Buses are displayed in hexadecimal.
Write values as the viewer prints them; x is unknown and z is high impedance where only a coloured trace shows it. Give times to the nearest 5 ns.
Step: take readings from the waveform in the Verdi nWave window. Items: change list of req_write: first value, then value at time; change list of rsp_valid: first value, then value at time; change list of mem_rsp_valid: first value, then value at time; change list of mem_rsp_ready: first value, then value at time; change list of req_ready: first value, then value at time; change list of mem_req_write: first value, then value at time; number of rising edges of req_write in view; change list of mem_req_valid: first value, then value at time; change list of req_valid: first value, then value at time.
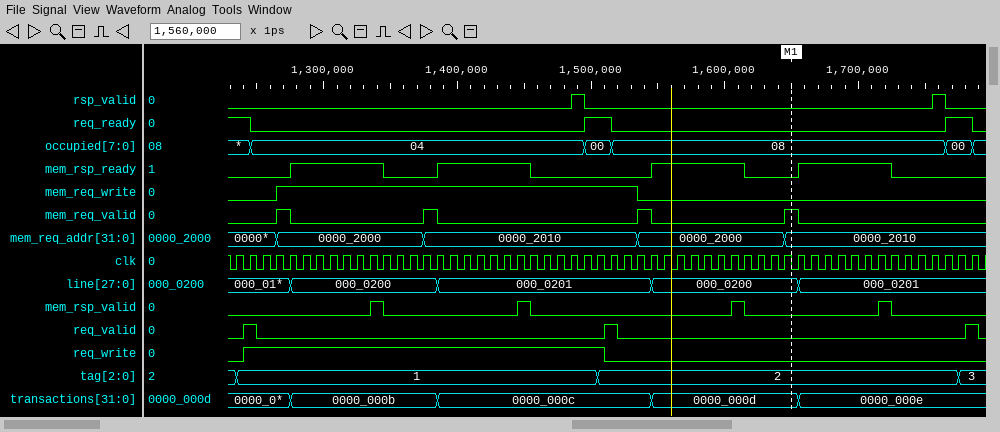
0, 1 at 1240 ns, 0 at 1510 ns
0, 1 at 1485 ns, 0 at 1495 ns, 1 at 1755 ns, 0 at 1765 ns
0, 1 at 1335 ns, 0 at 1345 ns, 1 at 1445 ns, 0 at 1455 ns, 1 at 1605 ns, 0 at 1615 ns, 1 at 1715 ns, 0 at 1725 ns
0, 1 at 1275 ns, 0 at 1345 ns, 1 at 1385 ns, 0 at 1455 ns, 1 at 1545 ns, 0 at 1615 ns, 1 at 1655 ns, 0 at 1725 ns
1, 0 at 1245 ns, 1 at 1495 ns, 0 at 1515 ns, 1 at 1765 ns, 0 at 1785 ns
0, 1 at 1265 ns, 0 at 1535 ns
1
0, 1 at 1265 ns, 0 at 1275 ns, 1 at 1375 ns, 0 at 1385 ns, 1 at 1535 ns, 0 at 1545 ns, 1 at 1645 ns, 0 at 1655 ns
0, 1 at 1240 ns, 0 at 1250 ns, 1 at 1510 ns, 0 at 1520 ns, 1 at 1780 ns, 0 at 1790 ns
